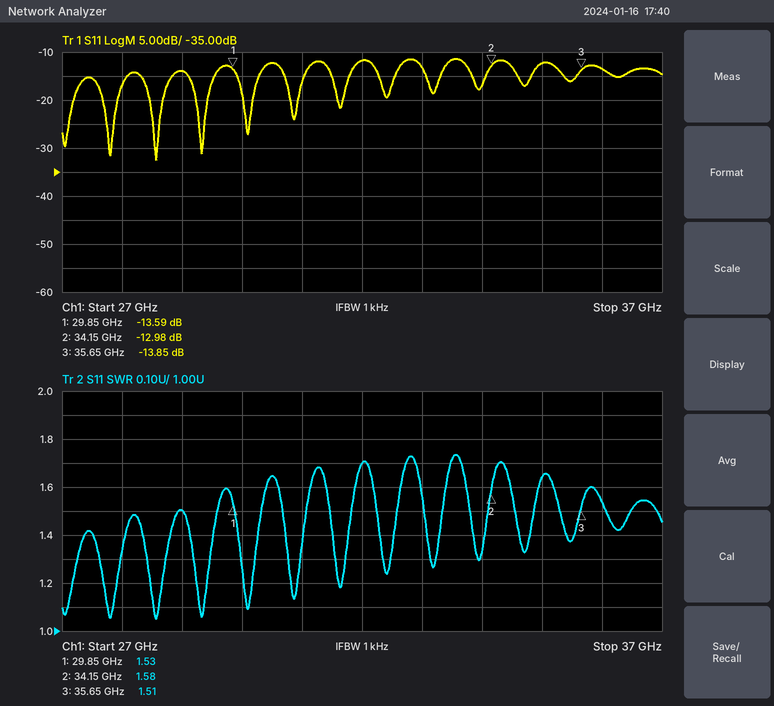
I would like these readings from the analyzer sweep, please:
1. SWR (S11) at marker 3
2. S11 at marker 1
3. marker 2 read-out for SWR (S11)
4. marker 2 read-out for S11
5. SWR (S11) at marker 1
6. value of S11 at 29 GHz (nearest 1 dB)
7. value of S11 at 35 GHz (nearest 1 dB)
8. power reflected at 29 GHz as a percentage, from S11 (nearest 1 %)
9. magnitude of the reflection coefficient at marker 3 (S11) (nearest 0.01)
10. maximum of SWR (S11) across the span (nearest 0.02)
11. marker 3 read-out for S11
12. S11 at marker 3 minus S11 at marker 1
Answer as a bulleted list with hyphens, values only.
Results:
- 1.51
- -13.59 dB
- 1.58
- -12.98 dB
- 1.53
- -14 dB
- -12 dB
- 4 %
- 0.20
- 1.74
- -13.85 dB
- -0.26 dB
